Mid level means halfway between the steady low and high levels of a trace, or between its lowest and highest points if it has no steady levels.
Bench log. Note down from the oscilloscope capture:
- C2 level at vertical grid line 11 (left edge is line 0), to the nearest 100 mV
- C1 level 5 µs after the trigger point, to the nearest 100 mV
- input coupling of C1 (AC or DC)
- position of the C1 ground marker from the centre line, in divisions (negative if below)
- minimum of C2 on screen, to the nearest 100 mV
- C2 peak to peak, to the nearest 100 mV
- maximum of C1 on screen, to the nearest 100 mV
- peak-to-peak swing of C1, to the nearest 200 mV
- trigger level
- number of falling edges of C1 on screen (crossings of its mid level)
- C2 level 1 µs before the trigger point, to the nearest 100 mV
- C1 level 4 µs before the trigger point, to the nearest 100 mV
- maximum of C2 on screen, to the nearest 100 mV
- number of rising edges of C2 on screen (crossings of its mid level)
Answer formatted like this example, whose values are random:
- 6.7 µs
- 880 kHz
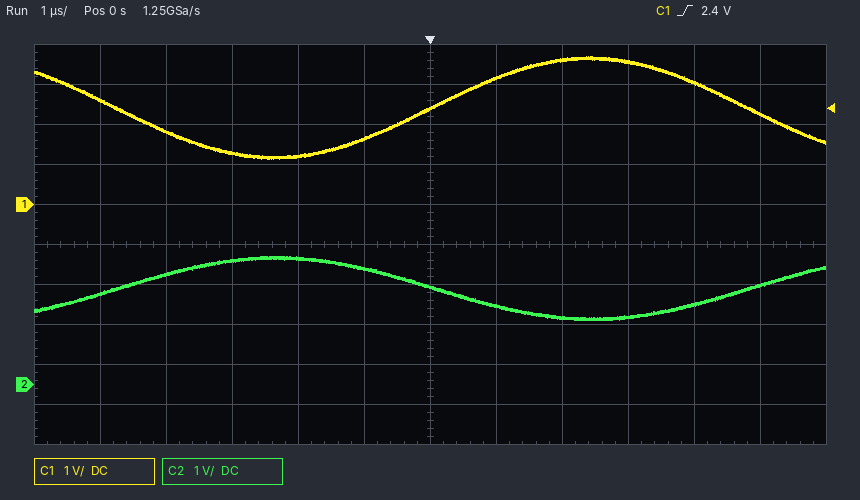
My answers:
- 2.5 V
- 2.3 V
- DC
- +1.0 div
- 1.6 V
- 1.6 V
- 3.7 V
- 2.6 V
- 2.4 V
- 2
- 2.9 V
- 1.8 V
- 3.2 V
- 2
